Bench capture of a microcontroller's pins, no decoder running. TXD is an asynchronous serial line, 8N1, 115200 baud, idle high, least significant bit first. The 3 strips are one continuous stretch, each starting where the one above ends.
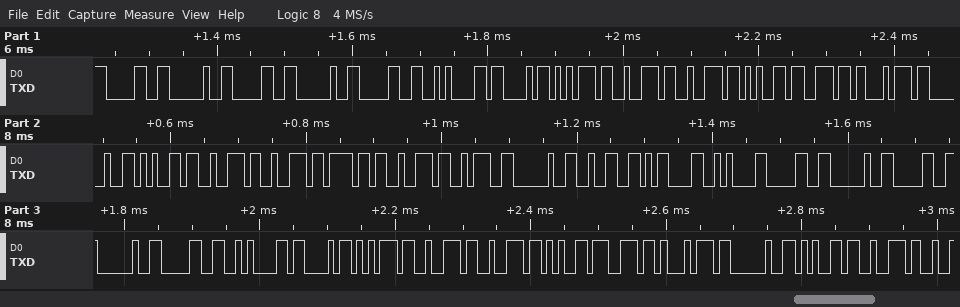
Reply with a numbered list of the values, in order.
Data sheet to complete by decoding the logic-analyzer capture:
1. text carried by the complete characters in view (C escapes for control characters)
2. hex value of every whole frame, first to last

1. "0 0 0\nCurrent error: 2\r\n0 0 0\nCurrent er"
2. 30 20 30 20 30 0A 43 75 72 72 65 6E 74 20 65 72 72 6F 72 3A 20 32 0D 0A 30 20 30 20 30 0A 43 75 72 72 65 6E 74 20 65 72
